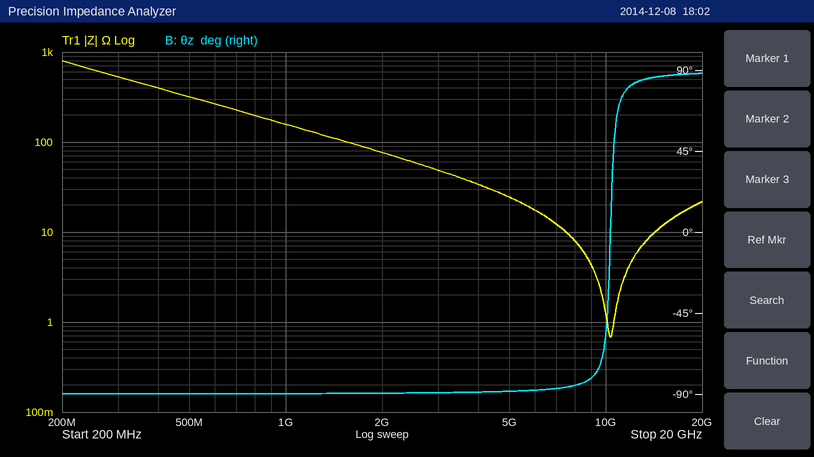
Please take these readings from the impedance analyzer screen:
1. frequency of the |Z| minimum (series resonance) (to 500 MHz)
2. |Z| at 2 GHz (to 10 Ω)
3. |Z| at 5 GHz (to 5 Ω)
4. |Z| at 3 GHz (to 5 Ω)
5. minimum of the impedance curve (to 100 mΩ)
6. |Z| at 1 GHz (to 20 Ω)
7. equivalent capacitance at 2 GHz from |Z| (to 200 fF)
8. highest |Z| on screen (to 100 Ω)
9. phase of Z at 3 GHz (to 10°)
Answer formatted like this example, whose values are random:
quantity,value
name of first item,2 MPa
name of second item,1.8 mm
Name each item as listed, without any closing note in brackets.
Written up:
quantity,value
frequency of the |Z| minimum (series resonance),10.5 GHz
|Z| at 2 GHz,80 Ω
|Z| at 5 GHz,25 Ω
|Z| at 3 GHz,50 Ω
minimum of the impedance curve,700 mΩ
|Z| at 1 GHz,160 Ω
equivalent capacitance at 2 GHz from |Z|,1.0 pF
highest |Z| on screen,800 Ω
phase of Z at 3 GHz,-90°
